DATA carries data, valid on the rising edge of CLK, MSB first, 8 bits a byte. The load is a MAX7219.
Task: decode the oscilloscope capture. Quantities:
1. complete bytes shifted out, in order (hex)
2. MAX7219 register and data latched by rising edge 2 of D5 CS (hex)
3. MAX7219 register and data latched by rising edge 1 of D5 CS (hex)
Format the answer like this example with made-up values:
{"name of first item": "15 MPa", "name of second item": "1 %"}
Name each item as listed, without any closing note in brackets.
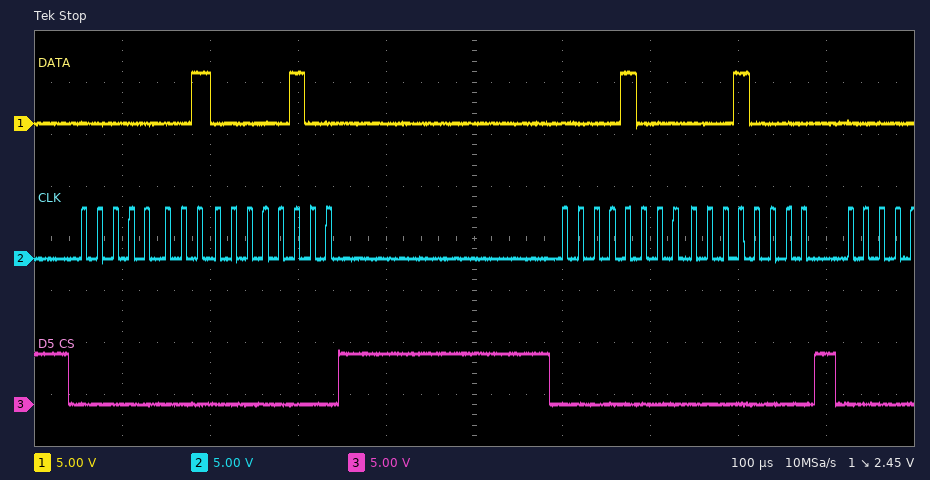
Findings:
{"complete bytes shifted out, in order": "01 04 08 10", "MAX7219 register and data latched by rising edge 2 of D5 CS": "register 0x8, data 0x10", "MAX7219 register and data latched by rising edge 1 of D5 CS": "register 0x1, data 0x04"}
